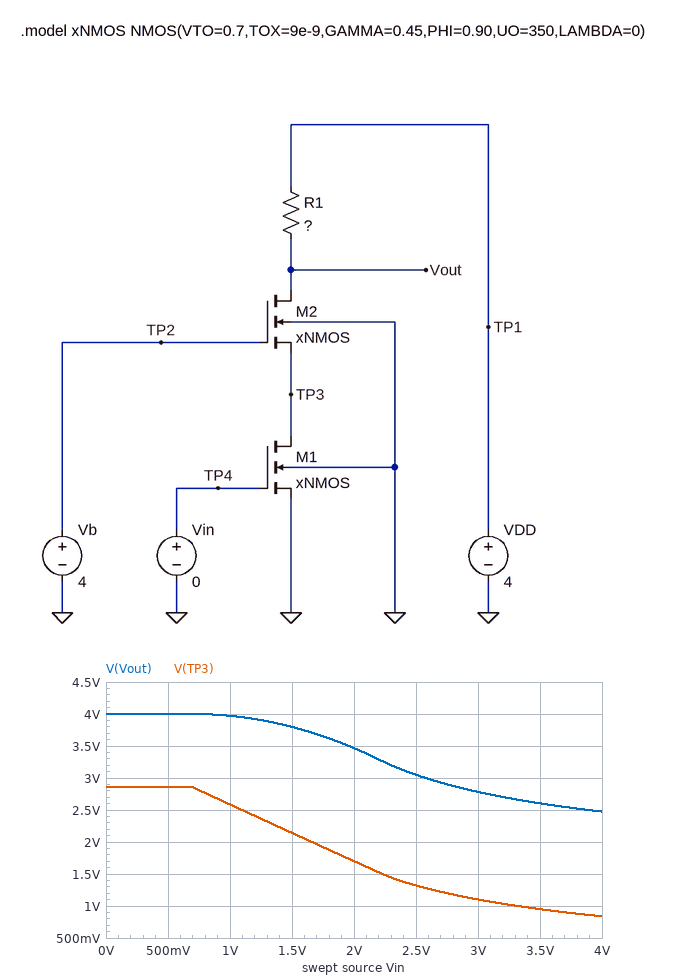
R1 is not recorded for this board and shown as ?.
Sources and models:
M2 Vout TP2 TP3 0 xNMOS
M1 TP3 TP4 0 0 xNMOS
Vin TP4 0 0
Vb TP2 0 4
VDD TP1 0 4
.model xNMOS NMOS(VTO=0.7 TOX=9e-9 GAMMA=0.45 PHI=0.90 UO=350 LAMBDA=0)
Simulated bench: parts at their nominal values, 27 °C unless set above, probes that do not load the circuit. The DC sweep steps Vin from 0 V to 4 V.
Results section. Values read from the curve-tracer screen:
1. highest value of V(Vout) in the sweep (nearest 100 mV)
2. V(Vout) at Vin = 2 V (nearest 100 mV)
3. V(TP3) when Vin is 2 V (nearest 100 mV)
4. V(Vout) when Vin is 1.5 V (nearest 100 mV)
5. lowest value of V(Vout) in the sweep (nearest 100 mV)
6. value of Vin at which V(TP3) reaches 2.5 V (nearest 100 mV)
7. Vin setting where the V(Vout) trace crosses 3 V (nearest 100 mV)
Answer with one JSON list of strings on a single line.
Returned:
["4.0 V", "3.5 V", "1.7 V", "3.8 V", "2.5 V", "1.1 V", "2.6 V"]
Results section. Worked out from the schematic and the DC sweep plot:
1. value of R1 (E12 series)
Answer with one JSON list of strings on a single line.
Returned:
["4.7 kΩ"]
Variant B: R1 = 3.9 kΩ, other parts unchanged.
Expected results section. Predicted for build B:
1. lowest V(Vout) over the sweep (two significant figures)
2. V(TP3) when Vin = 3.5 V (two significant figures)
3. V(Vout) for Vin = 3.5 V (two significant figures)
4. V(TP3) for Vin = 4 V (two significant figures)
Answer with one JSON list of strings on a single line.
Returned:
["2.7 V", "970 mV", "2.8 V", "860 mV"]
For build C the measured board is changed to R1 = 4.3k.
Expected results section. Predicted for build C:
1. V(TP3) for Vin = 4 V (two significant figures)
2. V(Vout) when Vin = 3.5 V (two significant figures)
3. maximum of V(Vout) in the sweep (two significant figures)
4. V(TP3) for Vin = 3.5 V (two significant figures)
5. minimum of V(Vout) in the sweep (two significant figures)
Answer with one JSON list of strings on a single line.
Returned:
["850 mV", "2.7 V", "4.0 V", "960 mV", "2.6 V"]
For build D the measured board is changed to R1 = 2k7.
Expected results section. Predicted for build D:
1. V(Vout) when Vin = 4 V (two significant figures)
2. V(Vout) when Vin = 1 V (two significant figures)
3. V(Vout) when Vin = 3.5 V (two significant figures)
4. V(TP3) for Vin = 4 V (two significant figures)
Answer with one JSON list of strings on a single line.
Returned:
["3.1 V", "4.0 V", "3.2 V", "880 mV"]
